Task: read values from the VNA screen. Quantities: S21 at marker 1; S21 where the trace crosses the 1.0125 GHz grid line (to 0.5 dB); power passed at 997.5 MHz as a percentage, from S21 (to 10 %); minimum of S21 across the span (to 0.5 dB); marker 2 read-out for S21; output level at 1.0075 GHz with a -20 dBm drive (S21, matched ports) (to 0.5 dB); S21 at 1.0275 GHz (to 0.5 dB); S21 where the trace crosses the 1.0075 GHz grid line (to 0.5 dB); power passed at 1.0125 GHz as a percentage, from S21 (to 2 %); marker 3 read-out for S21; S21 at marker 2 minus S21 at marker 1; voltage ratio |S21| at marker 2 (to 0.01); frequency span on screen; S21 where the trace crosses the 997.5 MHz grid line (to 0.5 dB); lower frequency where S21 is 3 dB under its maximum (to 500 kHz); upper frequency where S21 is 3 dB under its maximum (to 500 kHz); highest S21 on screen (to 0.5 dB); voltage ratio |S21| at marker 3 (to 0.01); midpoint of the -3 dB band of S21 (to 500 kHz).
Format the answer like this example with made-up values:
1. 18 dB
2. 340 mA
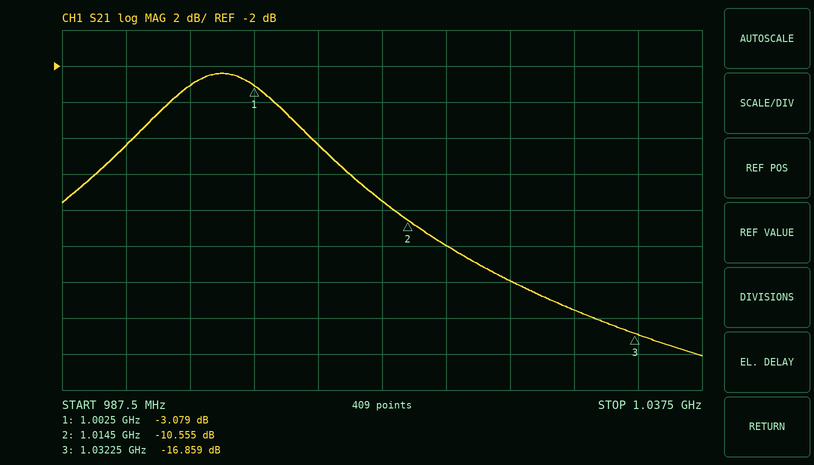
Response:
1. -3.079 dB
2. -9.5 dB
3. 50 %
4. -18.0 dB
5. -10.555 dB
6. -26.5 dBm
7. -15.5 dB
8. -6.5 dB
9. 12 %
10. -16.859 dB
11. -7.476 dB
12. 0.30
13. 50 MHz
14. -3.0 dB
15. 994.0 MHz
16. 1.0060 GHz
17. -2.5 dB
18. 0.14
19. 1.0000 GHz
